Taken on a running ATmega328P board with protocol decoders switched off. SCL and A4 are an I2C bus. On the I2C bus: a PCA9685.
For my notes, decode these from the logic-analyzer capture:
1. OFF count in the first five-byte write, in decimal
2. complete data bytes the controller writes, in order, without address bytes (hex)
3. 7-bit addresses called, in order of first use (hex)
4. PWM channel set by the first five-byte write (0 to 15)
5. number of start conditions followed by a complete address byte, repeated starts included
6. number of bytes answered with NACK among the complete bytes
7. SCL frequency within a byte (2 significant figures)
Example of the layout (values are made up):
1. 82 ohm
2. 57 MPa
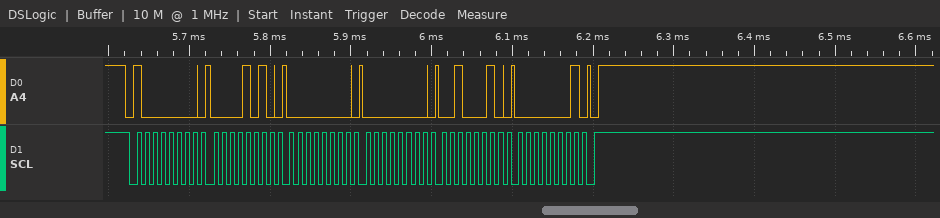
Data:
1. 290
2. 0A 00 00 22 01
3. 0x40
4. 1
5. 1
6. 0
7. 100 kHz
